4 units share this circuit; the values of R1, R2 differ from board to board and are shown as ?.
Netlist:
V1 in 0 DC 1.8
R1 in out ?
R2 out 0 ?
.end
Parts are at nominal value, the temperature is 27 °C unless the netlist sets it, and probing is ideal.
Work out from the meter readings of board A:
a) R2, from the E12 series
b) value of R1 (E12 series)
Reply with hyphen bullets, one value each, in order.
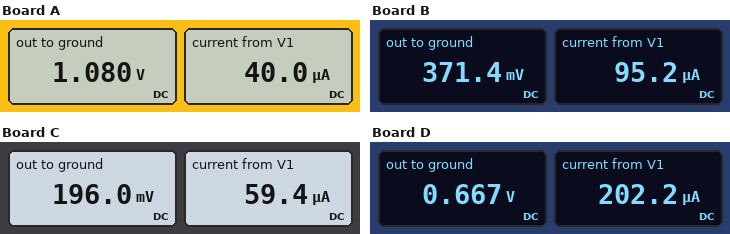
- 27 kΩ
- 18 kΩ
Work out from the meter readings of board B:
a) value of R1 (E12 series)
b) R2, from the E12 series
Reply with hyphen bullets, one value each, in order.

- 15 kΩ
- 3.9 kΩ
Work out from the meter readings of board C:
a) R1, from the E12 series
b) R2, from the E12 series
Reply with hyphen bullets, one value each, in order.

- 27 kΩ
- 3.3 kΩ
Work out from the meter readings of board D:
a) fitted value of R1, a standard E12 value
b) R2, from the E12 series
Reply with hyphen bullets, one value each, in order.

- 5.6 kΩ
- 3.3 kΩ
